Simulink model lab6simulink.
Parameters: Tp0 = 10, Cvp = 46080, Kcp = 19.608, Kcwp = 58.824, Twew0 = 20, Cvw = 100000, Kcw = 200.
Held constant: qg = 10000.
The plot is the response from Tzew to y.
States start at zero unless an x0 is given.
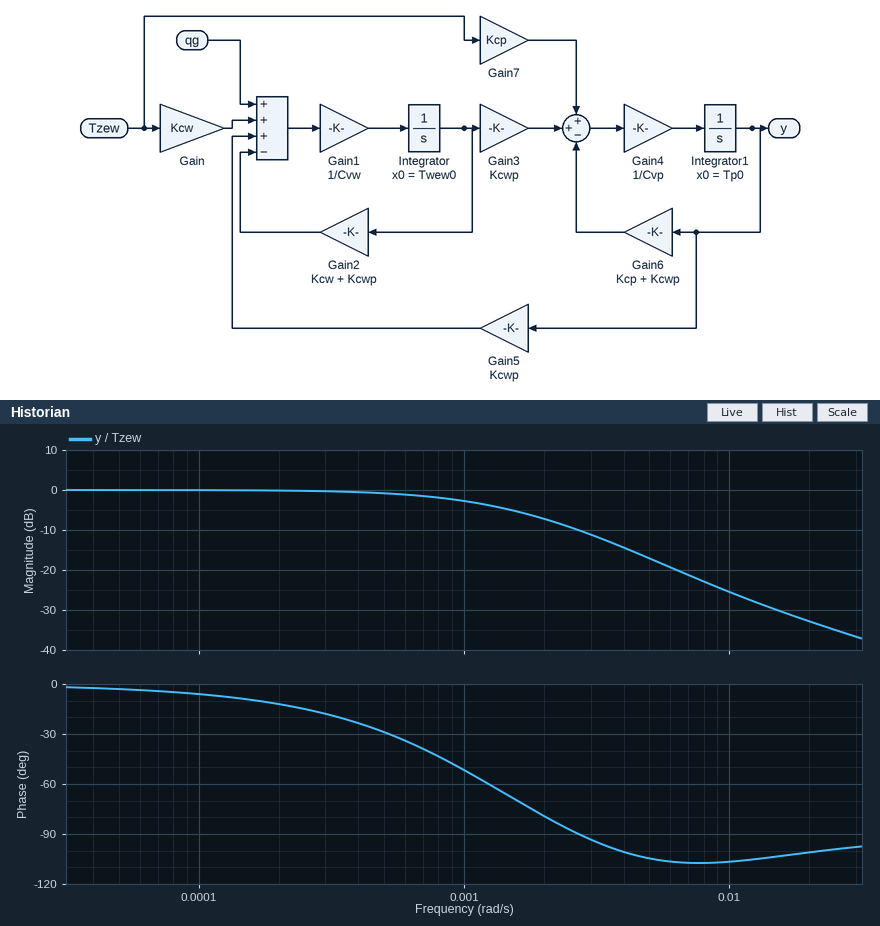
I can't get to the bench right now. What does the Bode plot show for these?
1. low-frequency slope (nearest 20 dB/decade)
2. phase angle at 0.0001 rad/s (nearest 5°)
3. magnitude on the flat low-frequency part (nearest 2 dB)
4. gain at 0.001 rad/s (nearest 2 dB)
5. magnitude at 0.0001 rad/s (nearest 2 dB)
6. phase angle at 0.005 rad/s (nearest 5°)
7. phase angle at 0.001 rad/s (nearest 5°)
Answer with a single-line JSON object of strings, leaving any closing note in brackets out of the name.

{"low-frequency slope": "0 dB/decade", "phase angle at 0.0001 rad/s": "-5°", "magnitude on the flat low-frequency part": "0 dB", "gain at 0.001 rad/s": "-2 dB", "magnitude at 0.0001 rad/s": "0 dB", "phase angle at 0.005 rad/s": "-105°", "phase angle at 0.001 rad/s": "-50°"}
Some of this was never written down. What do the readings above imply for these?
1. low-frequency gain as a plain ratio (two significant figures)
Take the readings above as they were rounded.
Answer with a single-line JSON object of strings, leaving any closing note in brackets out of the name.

{"low-frequency gain as a plain ratio": "1.0"}
